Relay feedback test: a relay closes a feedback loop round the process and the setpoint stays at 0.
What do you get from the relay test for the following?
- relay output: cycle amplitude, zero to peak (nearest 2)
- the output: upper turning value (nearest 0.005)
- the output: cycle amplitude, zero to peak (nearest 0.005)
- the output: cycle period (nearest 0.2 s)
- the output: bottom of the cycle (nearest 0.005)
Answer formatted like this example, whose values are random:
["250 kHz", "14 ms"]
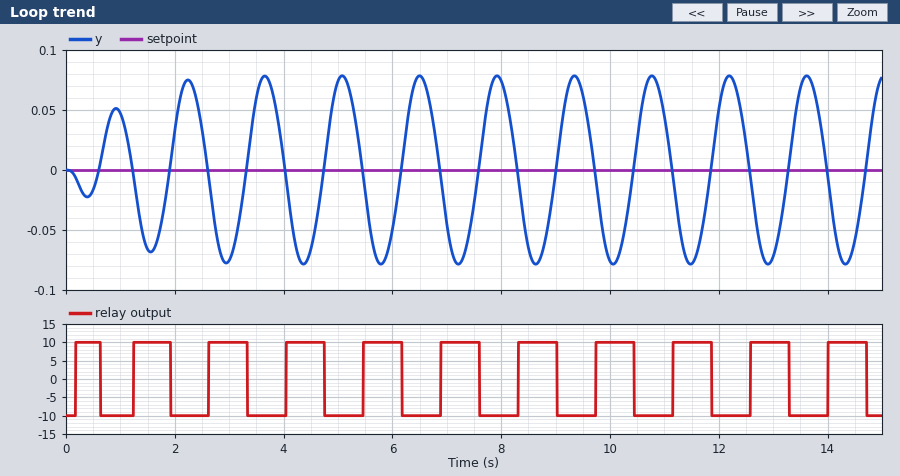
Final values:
["10", "0.080", "0.080", "1.4 s", "-0.080"]
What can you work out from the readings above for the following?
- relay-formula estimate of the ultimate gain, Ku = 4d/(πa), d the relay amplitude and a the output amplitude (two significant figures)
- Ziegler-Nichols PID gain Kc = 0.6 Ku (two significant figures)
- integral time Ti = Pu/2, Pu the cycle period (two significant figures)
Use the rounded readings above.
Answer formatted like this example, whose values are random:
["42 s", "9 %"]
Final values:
["160", "96", "0.70 s"]
